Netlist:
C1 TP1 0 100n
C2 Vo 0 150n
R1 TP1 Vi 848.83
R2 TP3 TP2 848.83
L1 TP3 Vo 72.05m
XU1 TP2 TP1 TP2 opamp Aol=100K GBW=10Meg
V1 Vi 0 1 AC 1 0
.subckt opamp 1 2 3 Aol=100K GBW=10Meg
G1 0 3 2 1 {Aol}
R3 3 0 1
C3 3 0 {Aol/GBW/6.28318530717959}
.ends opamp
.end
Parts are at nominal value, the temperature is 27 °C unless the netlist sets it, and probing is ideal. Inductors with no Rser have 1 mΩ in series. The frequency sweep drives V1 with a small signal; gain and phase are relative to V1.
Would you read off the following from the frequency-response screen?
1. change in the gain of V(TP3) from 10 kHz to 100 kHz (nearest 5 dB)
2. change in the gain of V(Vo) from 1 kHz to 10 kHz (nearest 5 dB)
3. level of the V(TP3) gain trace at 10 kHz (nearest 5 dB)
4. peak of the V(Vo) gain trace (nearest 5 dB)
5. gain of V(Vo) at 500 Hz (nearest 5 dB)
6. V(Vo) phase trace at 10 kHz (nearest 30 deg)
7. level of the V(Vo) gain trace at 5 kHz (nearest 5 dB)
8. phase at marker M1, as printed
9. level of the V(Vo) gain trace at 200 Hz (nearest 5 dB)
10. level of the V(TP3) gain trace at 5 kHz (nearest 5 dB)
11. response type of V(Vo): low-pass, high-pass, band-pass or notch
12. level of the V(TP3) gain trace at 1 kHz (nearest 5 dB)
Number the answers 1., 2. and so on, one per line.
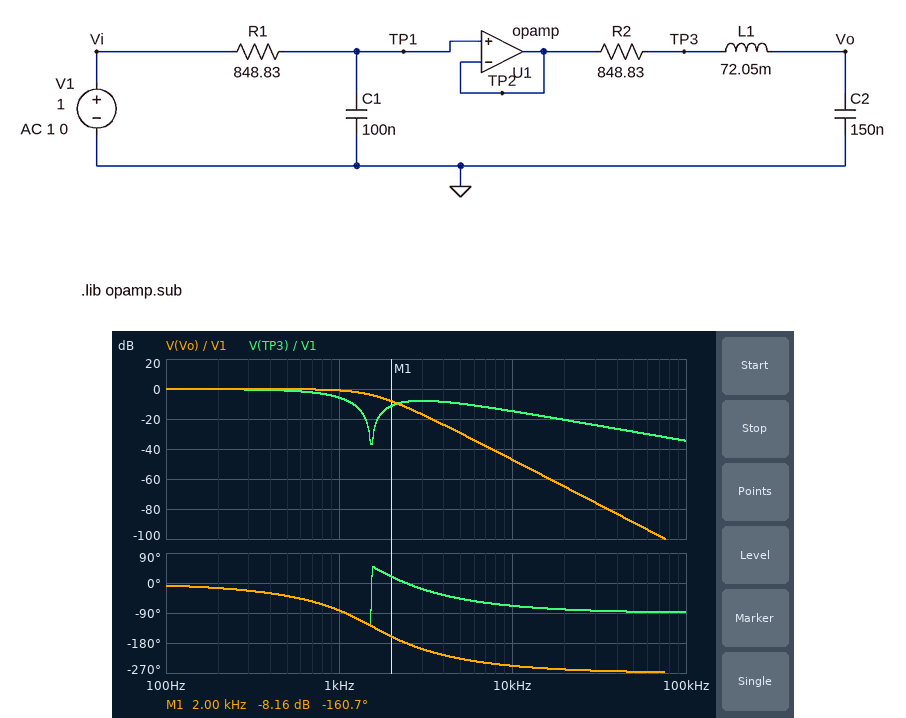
1. -20 dB
2. -45 dB
3. -15 dB
4. 0 dB
5. 0 dB
6. -240 deg
7. -30 dB
8. -160.7 deg
9. 0 dB
10. -10 dB
11. low-pass
12. -5 dB
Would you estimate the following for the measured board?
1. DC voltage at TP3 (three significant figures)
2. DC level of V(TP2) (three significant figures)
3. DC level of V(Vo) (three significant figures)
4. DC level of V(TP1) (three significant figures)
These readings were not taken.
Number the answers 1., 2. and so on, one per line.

1. 1.00 V
2. 1.00 V
3. 1.00 V
4. 1.00 V
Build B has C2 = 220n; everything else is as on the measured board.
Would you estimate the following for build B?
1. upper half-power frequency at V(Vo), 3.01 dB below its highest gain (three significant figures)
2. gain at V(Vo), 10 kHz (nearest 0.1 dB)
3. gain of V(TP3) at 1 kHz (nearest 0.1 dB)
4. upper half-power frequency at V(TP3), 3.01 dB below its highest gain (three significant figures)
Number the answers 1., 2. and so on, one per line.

1. 1.02 kHz
2. -50.6 dB
3. -11.4 dB
4. 598 Hz
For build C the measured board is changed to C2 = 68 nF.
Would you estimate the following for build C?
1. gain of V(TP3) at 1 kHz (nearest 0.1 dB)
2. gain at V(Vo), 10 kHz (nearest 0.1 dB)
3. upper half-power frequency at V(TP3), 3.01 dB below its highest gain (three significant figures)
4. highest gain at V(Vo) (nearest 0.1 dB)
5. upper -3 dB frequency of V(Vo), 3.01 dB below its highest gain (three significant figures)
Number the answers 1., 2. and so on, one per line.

1. -1.9 dB
2. -40.1 dB
3. 1.23 kHz
4. 0 dB
5. 2.39 kHz
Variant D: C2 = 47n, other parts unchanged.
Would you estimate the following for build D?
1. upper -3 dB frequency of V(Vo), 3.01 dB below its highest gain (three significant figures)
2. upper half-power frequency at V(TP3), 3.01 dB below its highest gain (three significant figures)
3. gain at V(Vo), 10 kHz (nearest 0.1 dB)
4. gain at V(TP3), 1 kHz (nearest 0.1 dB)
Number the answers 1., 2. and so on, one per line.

1. 2.95 kHz
2. 1.45 kHz
3. -36.7 dB
4. -1.4 dB
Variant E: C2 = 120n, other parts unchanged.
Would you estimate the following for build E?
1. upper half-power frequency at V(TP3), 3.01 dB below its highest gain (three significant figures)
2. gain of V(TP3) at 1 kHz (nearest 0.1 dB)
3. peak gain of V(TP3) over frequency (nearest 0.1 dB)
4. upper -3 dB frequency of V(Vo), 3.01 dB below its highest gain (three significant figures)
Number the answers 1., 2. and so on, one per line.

1. 897 Hz
2. -4.0 dB
3. 0 dB
4. 1.65 kHz
